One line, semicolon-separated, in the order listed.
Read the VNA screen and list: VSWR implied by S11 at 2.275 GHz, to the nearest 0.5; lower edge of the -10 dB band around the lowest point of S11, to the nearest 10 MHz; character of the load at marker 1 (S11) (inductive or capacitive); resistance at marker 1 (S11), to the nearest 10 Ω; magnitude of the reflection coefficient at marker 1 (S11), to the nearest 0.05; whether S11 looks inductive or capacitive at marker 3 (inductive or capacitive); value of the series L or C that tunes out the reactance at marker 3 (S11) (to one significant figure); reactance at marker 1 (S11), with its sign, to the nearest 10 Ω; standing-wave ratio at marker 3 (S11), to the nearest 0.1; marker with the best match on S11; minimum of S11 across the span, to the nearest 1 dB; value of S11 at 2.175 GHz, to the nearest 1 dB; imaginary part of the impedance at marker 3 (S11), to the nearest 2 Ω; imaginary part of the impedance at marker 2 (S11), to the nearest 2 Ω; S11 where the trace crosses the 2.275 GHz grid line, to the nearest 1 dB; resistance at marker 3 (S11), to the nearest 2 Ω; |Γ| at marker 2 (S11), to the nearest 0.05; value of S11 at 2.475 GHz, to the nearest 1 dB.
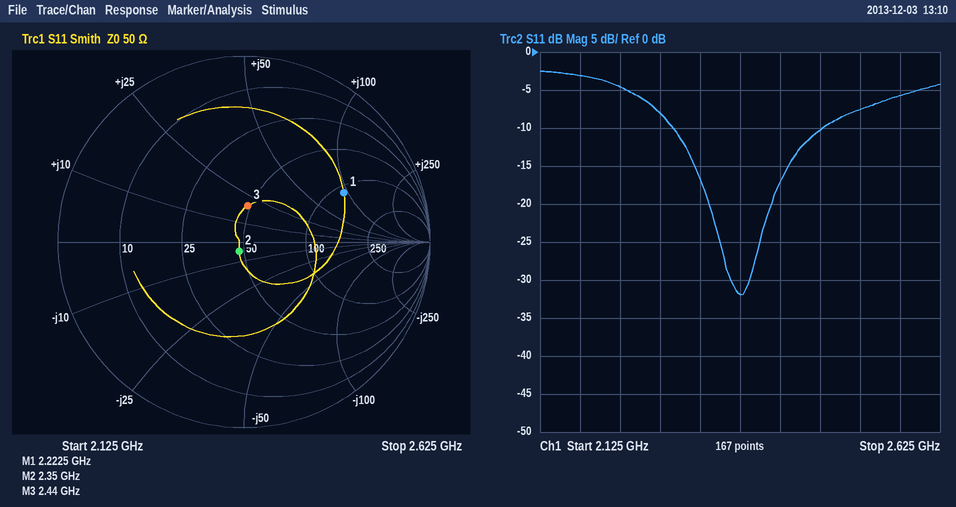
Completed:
2.5; 2.29 GHz; inductive; 110 Ω; 0.60; inductive; 3 pF; +90 Ω; 1.5; marker 2; -32 dB; -3 dB; +20 Ω; -4 Ω; -8 dB; 48 Ω; 0.05; -10 dB
